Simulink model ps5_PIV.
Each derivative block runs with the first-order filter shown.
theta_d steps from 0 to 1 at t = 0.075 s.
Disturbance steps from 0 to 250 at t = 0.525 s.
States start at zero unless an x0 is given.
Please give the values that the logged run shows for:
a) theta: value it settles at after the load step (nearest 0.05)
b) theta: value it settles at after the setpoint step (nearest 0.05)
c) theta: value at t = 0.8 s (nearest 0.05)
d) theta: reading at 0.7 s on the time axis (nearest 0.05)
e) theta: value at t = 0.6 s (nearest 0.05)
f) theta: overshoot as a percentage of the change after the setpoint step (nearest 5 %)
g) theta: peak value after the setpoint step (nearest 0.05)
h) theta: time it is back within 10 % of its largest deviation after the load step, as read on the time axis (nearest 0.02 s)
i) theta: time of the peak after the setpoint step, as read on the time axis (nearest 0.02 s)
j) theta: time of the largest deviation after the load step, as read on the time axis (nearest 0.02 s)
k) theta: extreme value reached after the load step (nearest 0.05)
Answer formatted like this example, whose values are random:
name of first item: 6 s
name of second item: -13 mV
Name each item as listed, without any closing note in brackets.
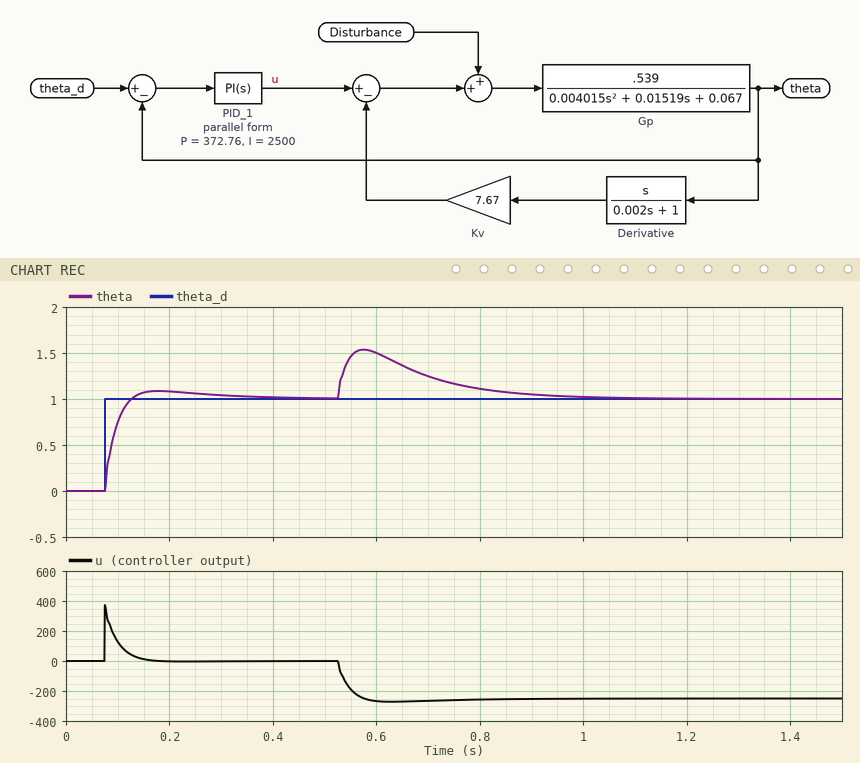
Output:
theta: value it settles at after the load step: 1.00
theta: value it settles at after the setpoint step: 1.00
theta: value at t = 0.8 s: 1.10
theta: reading at 0.7 s on the time axis: 1.25
theta: value at t = 0.6 s: 1.50
theta: overshoot as a percentage of the change after the setpoint step: 10 %
theta: peak value after the setpoint step: 1.10
theta: time it is back within 10 % of its largest deviation after the load step, as read on the time axis: 0.90 s
theta: time of the peak after the setpoint step, as read on the time axis: 0.18 s
theta: time of the largest deviation after the load step, as read on the time axis: 0.58 s
theta: extreme value reached after the load step: 1.55
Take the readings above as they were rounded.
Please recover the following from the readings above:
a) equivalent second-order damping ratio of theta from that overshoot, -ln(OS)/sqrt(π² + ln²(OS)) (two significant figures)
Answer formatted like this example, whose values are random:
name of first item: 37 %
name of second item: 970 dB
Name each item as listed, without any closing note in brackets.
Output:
equivalent second-order damping ratio of theta from that overshoot, -ln(OS)/sqrt(π² + ln²(OS)): 0.59
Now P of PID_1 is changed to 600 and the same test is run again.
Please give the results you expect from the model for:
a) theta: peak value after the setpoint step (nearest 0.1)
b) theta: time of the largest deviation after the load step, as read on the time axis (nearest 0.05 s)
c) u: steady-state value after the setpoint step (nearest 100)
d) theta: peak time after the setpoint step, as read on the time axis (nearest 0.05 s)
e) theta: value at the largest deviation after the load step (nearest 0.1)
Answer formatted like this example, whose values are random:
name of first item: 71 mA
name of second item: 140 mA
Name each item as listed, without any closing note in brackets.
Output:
theta: peak value after the setpoint step: 1.0
theta: time of the largest deviation after the load step, as read on the time axis: 0.55 s
u: steady-state value after the setpoint step: 0
theta: peak time after the setpoint step, as read on the time axis: 0.15 s
theta: value at the largest deviation after the load step: 1.4
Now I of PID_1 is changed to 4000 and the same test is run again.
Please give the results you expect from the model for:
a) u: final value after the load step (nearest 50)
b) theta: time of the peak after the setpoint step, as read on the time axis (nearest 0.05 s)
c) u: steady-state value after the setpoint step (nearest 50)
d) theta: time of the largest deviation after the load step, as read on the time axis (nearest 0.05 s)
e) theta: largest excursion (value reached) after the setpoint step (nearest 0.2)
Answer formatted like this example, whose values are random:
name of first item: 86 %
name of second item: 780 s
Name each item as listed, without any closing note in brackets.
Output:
u: final value after the load step: -250
theta: time of the peak after the setpoint step, as read on the time axis: 0.15 s
u: steady-state value after the setpoint step: 0
theta: time of the largest deviation after the load step, as read on the time axis: 0.55 s
theta: largest excursion (value reached) after the setpoint step: 1.2
